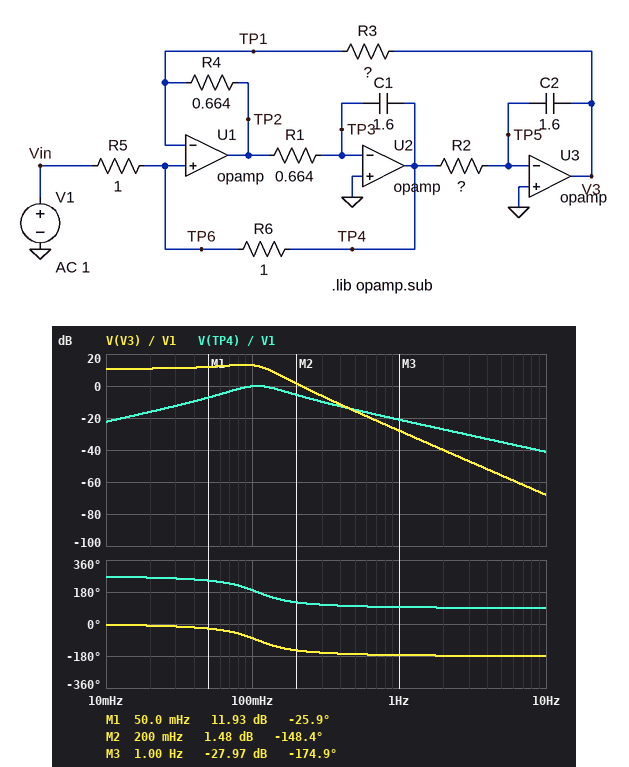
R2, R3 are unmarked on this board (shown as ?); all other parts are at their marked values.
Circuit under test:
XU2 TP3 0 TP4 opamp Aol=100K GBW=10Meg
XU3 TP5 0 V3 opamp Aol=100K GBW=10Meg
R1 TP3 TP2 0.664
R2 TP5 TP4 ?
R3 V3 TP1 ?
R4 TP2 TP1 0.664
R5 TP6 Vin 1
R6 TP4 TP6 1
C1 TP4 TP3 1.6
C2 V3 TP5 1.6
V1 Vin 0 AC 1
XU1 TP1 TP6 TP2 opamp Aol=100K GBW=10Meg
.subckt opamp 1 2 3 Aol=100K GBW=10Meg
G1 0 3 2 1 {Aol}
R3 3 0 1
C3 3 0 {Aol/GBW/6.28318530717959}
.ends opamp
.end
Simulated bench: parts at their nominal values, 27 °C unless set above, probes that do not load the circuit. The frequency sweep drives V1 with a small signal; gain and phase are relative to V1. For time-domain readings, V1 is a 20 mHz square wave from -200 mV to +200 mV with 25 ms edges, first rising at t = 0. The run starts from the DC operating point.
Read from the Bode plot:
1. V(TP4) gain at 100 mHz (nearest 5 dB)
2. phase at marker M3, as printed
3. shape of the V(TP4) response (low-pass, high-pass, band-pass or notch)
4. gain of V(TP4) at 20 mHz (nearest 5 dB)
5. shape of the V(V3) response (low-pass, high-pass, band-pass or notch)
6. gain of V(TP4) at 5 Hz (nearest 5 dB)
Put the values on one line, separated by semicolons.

0 dB; -174.9 deg; band-pass; -15 dB; low-pass; -35 dB
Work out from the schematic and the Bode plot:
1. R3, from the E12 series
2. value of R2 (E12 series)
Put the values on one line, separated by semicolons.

3.9 Ω; 0.22 Ω
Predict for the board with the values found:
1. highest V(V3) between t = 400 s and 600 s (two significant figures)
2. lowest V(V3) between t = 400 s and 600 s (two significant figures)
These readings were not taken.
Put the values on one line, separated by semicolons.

1.0 V; -1.0 V
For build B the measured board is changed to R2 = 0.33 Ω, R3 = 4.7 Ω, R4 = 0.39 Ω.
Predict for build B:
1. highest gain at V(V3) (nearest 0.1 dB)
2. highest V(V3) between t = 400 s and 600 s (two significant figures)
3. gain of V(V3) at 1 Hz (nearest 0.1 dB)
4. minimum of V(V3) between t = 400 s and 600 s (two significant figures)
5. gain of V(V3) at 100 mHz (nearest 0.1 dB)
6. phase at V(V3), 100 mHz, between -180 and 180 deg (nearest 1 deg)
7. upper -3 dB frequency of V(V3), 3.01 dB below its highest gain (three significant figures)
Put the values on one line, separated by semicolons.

16.4 dB; 1.5 V; -32.2 dB; -1.5 V; 7.6 dB; -128 deg; 64.6 mHz
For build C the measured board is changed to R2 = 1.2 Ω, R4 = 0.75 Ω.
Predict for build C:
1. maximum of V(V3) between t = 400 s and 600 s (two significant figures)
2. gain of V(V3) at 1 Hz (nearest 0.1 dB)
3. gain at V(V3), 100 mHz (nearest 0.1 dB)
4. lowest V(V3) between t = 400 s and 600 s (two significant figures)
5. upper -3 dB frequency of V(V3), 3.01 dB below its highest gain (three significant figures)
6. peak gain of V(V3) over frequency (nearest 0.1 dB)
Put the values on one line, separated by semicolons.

620 mV; -42.6 dB; -4.0 dB; -620 mV; 35.7 mHz; 9.8 dB
